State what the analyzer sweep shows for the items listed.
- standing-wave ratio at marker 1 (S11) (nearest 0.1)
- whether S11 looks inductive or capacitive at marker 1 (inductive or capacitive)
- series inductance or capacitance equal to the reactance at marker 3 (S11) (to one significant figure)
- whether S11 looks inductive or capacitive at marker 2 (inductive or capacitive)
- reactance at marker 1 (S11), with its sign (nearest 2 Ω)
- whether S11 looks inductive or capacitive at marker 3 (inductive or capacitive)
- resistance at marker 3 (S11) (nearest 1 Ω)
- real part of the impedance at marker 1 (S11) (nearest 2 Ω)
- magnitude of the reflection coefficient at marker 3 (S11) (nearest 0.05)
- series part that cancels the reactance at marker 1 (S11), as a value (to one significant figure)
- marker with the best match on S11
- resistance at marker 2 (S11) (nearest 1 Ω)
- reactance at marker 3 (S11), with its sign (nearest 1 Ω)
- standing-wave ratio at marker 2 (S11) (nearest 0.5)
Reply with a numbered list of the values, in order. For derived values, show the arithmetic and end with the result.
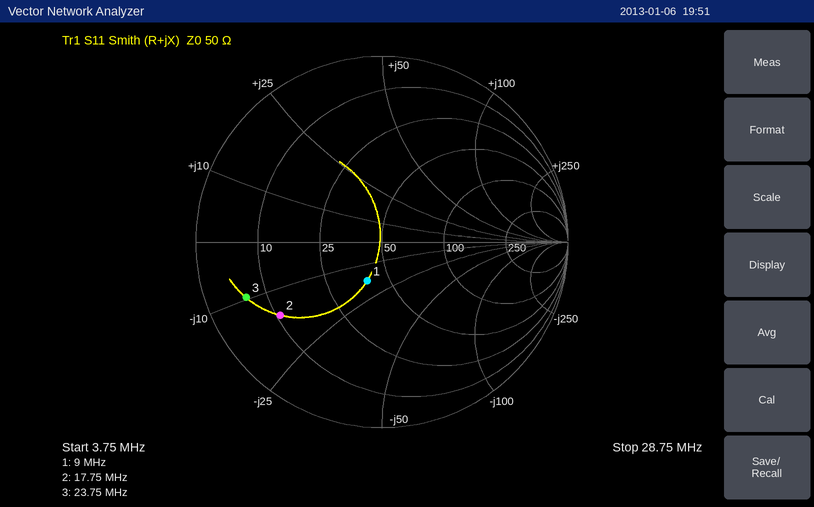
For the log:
1. 1.6
2. capacitive
3. C = 1/(2π × 23.75 MHz × 10 Ω) ≈ 670 pF, so 700 pF to one significant figure
4. capacitive
5. -18 Ω
6. capacitive
7. 6 Ω
8. 40 Ω
9. 0.80
10. L = 18 Ω/(2π × 9 MHz) ≈ 318 nH, so 300 nH to one significant figure
11. marker 1
12. 11 Ω
13. -10 Ω
14. 5.0
